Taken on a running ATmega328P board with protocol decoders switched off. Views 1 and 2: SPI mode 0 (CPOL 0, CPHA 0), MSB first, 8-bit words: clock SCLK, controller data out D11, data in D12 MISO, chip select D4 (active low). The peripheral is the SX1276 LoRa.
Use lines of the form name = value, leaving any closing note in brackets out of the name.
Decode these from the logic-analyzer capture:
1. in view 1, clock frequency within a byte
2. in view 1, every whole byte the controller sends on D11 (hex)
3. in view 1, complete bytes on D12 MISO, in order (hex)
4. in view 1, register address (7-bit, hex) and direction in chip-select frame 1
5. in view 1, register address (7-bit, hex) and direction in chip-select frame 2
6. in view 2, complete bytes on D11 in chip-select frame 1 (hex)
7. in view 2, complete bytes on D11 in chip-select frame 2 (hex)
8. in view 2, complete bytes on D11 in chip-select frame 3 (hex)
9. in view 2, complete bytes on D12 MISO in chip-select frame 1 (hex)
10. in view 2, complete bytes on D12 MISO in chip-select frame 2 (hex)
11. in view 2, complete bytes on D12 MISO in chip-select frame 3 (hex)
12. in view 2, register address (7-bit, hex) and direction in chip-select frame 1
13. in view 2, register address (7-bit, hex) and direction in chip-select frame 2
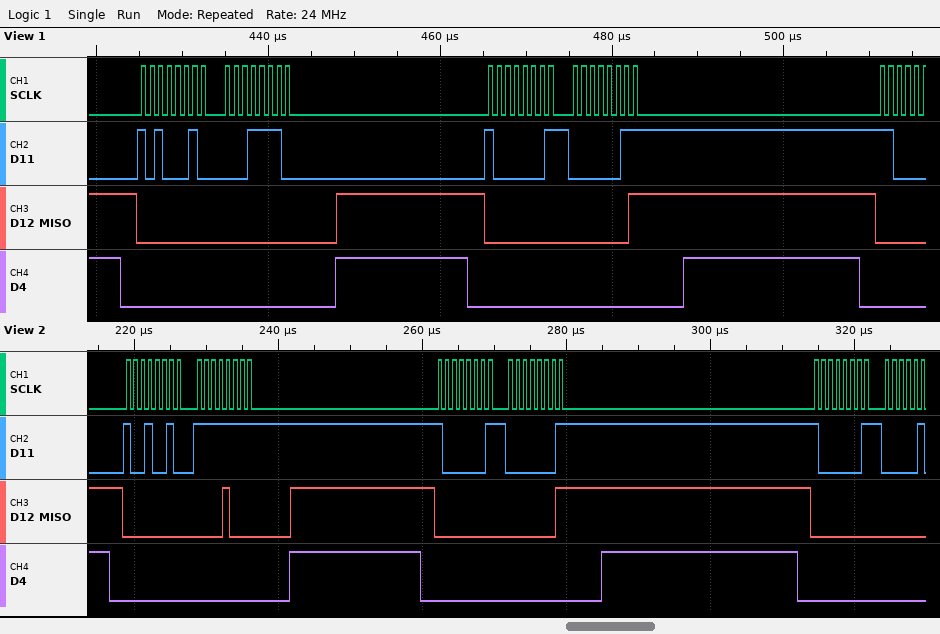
in view 1, clock frequency within a byte = 1 MHz
in view 1, every whole byte the controller sends on D11 = 0xA2 0x1E 0x81 0x03
in view 1, complete bytes on D12 MISO, in order = 0x00 0x00 0x00 0x01
in view 1, register address (7-bit, hex) and direction in chip-select frame 1 = 0x22 write
in view 1, register address (7-bit, hex) and direction in chip-select frame 2 = 0x01 write
in view 2, complete bytes on D11 in chip-select frame 1 = 0x92 0xFF
in view 2, complete bytes on D11 in chip-select frame 2 = 0x81 0x01
in view 2, complete bytes on D11 in chip-select frame 3 = 0x81
in view 2, complete bytes on D12 MISO in chip-select frame 1 = 0x00 0x08
in view 2, complete bytes on D12 MISO in chip-select frame 2 = 0x00 0x01
in view 2, complete bytes on D12 MISO in chip-select frame 3 = 0x00
in view 2, register address (7-bit, hex) and direction in chip-select frame 1 = 0x12 write
in view 2, register address (7-bit, hex) and direction in chip-select frame 2 = 0x01 write
